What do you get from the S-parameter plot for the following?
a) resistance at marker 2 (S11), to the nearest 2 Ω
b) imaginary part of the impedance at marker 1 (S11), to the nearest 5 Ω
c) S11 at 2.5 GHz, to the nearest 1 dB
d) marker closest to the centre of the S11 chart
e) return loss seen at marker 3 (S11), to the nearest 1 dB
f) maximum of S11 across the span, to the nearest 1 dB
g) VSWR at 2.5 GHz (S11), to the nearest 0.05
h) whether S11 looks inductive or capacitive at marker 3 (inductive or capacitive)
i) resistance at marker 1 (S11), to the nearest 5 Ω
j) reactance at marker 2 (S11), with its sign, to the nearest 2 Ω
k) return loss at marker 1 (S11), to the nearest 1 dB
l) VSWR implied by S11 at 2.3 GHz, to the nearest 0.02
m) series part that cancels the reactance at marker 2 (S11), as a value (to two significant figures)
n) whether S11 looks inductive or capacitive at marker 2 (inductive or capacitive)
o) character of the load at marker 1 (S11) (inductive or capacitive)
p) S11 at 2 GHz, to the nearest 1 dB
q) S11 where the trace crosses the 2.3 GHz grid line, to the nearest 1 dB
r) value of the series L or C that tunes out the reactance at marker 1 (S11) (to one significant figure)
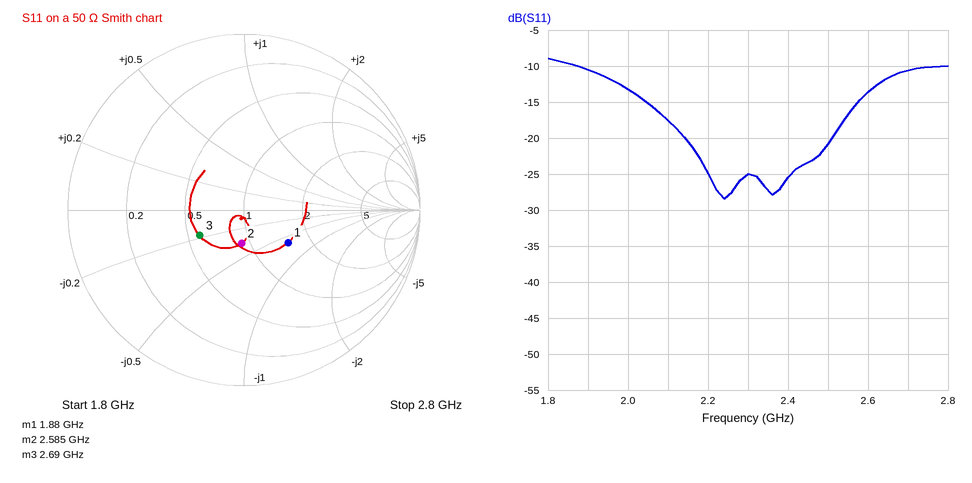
46 Ω
-30 Ω
-21 dB
marker 2
11 dB
-9 dB
1.20
capacitive
75 Ω
-18 Ω
10 dB
1.12
1.1 nH
capacitive
capacitive
-13 dB
-25 dB
3 nH
